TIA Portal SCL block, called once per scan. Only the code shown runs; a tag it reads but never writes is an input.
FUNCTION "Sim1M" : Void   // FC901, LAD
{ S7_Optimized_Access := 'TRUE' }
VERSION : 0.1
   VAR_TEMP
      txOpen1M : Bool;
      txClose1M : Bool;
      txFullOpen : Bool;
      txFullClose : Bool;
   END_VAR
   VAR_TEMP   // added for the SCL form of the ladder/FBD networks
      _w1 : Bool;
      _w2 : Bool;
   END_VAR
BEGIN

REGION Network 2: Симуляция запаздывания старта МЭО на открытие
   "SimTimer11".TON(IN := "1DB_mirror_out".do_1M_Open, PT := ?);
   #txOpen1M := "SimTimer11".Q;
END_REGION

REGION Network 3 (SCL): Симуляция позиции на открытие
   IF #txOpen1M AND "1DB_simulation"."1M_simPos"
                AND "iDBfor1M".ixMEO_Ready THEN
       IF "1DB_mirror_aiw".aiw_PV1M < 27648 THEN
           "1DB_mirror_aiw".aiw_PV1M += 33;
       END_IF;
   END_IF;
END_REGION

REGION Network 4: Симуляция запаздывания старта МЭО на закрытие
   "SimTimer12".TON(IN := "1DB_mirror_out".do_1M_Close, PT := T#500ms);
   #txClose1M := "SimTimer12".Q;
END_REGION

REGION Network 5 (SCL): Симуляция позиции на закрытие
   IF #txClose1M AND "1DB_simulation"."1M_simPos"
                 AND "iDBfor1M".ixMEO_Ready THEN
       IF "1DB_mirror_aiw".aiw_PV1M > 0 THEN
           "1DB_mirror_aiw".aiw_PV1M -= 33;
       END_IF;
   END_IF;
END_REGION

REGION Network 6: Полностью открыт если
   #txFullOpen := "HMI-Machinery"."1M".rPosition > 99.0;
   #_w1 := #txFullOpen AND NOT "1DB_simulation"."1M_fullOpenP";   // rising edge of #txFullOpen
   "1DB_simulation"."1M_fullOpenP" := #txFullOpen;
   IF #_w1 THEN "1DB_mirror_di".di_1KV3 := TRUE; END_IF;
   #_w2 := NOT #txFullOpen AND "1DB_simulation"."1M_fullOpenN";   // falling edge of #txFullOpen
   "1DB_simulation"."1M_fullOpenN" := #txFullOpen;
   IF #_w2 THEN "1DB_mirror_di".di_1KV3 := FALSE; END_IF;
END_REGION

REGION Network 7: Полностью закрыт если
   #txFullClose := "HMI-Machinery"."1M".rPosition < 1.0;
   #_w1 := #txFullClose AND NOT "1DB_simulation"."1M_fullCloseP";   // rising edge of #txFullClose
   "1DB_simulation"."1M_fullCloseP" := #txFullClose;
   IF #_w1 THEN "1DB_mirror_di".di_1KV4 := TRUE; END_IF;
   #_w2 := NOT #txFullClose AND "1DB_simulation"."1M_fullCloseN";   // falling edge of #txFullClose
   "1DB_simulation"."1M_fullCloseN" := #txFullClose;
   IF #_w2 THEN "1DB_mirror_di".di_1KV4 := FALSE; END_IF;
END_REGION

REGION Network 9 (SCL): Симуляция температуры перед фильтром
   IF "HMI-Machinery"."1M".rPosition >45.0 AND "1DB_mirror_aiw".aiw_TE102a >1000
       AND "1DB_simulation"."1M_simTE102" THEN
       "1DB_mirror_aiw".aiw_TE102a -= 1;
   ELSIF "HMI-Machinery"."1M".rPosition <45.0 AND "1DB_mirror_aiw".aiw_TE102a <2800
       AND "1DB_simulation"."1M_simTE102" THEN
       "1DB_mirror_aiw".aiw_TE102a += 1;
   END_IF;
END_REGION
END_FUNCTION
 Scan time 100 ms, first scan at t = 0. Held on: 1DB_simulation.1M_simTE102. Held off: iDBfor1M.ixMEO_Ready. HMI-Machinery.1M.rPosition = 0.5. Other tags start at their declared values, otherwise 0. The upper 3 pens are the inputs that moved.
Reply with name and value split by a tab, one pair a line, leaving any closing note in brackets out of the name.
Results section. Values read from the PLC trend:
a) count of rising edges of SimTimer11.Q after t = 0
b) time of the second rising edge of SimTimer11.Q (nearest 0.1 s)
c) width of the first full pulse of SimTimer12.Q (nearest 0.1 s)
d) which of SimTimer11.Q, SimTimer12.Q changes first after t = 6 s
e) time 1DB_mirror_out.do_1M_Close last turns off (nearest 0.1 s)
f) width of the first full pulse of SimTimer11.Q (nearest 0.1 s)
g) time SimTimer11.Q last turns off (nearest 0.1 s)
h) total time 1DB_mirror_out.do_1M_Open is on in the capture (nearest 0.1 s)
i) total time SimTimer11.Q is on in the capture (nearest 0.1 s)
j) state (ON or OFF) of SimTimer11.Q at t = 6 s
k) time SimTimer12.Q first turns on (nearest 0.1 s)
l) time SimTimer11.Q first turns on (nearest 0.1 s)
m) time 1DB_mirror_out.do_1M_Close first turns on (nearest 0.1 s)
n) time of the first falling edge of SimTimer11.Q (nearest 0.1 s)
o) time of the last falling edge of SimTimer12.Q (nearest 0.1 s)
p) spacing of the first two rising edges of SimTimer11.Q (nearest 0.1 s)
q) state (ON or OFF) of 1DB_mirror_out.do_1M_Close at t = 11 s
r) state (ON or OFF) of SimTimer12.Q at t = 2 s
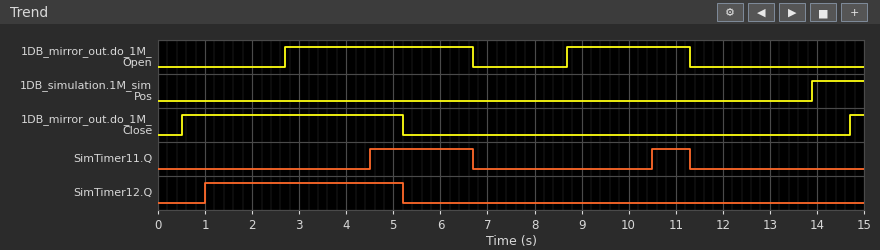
count of rising edges of SimTimer11.Q after t = 0	2
time of the second rising edge of SimTimer11.Q	10.5 s
width of the first full pulse of SimTimer12.Q	4.2 s
which of SimTimer11.Q, SimTimer12.Q changes first after t = 6 s	SimTimer11.Q
time 1DB_mirror_out.do_1M_Close last turns off	5.2 s
width of the first full pulse of SimTimer11.Q	2.2 s
time SimTimer11.Q last turns off	11.3 s
total time 1DB_mirror_out.do_1M_Open is on in the capture	6.6 s
total time SimTimer11.Q is on in the capture	3.0 s
state (ON or OFF) of SimTimer11.Q at t = 6 s	ON
time SimTimer12.Q first turns on	1.0 s
time SimTimer11.Q first turns on	4.5 s
time 1DB_mirror_out.do_1M_Close first turns on	0.5 s
time of the first falling edge of SimTimer11.Q	6.7 s
time of the last falling edge of SimTimer12.Q	5.2 s
spacing of the first two rising edges of SimTimer11.Q	6.0 s
state (ON or OFF) of 1DB_mirror_out.do_1M_Close at t = 11 s	OFF
state (ON or OFF) of SimTimer12.Q at t = 2 s	ON
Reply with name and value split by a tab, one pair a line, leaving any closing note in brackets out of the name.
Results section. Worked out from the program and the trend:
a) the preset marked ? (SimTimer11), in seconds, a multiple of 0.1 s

the preset marked ? (SimTimer11), in seconds, a multiple of 0.1 s	1.8 s
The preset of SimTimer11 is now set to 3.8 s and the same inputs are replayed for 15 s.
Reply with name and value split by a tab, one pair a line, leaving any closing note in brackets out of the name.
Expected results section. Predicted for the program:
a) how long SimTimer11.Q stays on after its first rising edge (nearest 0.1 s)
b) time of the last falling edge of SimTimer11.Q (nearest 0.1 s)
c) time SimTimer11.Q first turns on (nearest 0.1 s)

how long SimTimer11.Q stays on after its first rising edge	0.2 s
time of the last falling edge of SimTimer11.Q	6.7 s
time SimTimer11.Q first turns on	6.5 s
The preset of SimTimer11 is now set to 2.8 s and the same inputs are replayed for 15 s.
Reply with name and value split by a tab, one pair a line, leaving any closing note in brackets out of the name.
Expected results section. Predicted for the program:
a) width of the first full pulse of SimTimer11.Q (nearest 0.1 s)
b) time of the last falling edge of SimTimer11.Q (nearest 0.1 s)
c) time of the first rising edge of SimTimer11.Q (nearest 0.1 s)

width of the first full pulse of SimTimer11.Q	1.2 s
time of the last falling edge of SimTimer11.Q	6.7 s
time of the first rising edge of SimTimer11.Q	5.5 s
